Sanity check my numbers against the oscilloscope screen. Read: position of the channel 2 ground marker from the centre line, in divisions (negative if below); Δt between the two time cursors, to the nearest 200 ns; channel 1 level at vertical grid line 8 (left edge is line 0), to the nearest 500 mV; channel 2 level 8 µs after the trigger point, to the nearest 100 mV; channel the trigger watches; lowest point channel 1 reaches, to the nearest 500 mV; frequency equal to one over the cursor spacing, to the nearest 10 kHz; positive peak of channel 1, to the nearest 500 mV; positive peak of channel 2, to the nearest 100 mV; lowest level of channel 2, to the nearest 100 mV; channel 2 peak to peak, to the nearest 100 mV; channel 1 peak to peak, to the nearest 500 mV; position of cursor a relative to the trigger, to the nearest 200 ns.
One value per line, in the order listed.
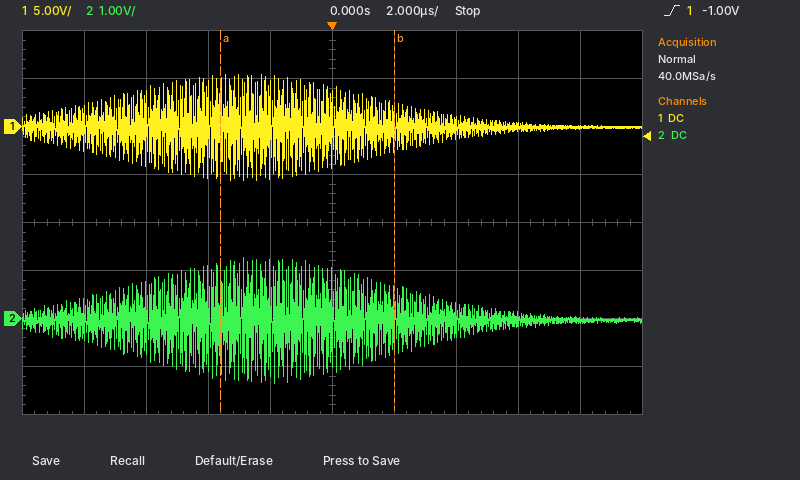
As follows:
-2.0 div
5.6 µs
0.0 V
0.0 V
channel 1
-5.5 V
180 kHz
5.5 V
1.3 V
-1.3 V
2.6 V
11.0 V
-3.6 µs
